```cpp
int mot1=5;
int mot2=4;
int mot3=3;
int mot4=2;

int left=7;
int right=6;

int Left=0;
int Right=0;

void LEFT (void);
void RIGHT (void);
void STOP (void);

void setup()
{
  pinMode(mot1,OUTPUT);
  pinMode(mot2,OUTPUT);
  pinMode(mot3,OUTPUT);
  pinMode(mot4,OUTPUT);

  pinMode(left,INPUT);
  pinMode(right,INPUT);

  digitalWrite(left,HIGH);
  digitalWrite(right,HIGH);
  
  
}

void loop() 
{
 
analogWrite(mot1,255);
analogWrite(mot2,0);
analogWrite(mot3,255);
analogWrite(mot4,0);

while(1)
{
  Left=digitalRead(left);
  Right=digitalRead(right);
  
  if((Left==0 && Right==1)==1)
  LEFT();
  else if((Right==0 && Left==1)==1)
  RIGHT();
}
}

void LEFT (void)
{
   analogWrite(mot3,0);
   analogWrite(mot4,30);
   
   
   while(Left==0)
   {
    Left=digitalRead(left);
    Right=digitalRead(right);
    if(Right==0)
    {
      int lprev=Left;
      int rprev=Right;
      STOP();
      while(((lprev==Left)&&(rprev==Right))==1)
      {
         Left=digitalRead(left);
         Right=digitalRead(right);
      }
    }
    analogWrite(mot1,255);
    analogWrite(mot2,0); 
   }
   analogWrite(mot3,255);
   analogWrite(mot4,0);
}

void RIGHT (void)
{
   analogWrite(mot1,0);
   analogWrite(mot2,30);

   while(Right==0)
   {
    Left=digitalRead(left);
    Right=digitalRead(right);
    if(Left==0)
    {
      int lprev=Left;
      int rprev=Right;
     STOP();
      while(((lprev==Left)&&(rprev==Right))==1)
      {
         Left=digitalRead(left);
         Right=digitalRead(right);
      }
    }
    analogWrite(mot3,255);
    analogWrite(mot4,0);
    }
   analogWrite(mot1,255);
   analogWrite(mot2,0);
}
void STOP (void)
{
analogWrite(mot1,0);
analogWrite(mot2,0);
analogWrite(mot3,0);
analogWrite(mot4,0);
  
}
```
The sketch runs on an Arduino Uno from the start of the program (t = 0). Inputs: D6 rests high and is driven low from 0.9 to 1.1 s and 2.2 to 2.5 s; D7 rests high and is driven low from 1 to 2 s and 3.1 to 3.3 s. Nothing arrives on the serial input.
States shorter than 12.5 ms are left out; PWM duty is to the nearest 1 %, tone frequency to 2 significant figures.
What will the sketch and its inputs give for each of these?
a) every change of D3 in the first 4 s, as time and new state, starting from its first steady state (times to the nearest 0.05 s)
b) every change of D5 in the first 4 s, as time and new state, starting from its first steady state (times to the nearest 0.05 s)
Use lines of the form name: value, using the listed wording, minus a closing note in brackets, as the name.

every change of D3 in the first 4 s, as time and new state, starting from its first steady state: 0 s high; 1 s low; 2 s high; 3.1 s low; 3.3 s high
every change of D5 in the first 4 s, as time and new state, starting from its first steady state: 0 s high; 0.9 s low; 1.1 s high; 2.2 s low; 2.5 s high
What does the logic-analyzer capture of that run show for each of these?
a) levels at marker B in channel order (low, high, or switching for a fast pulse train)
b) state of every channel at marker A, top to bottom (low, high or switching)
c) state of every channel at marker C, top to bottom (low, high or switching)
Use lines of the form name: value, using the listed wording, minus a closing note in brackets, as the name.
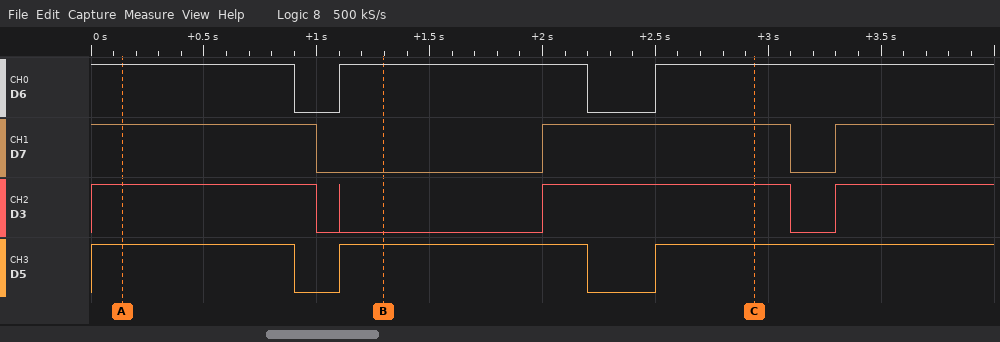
levels at marker B in channel order: D6 high, D7 low, D3 low, D5 high
state of every channel at marker A, top to bottom: D6 high, D7 high, D3 high, D5 high
state of every channel at marker C, top to bottom: D6 high, D7 high, D3 high, D5 high
